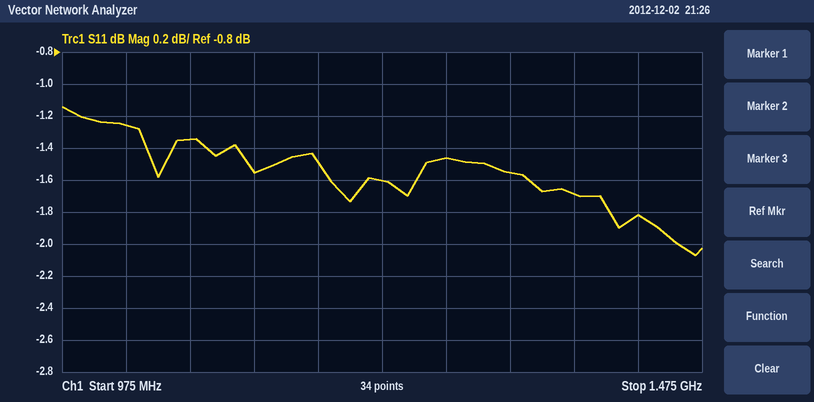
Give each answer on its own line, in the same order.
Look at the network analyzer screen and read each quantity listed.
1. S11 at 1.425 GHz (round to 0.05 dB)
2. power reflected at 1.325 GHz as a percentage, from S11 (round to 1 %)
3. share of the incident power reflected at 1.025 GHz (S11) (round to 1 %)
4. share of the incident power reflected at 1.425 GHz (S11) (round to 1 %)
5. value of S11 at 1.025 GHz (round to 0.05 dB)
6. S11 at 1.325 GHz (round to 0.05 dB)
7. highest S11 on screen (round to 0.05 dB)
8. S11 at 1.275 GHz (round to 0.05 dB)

-1.80 dB
70 %
75 %
66 %
-1.25 dB
-1.55 dB
-1.15 dB
-1.45 dB
